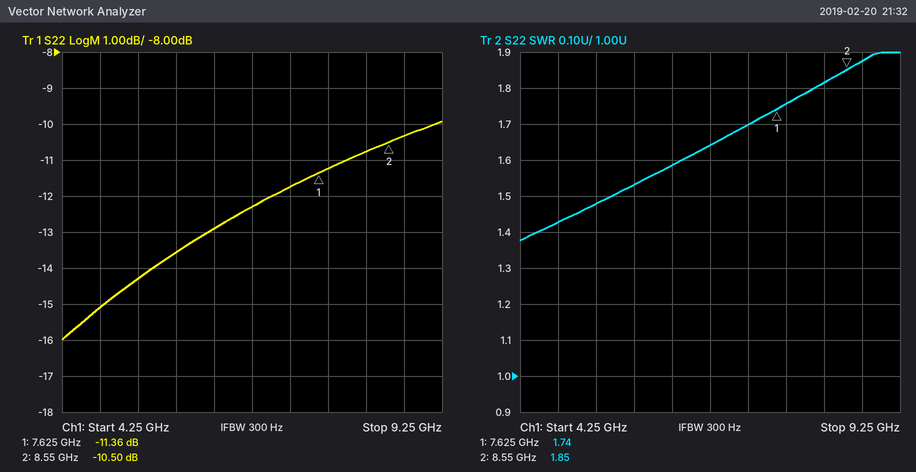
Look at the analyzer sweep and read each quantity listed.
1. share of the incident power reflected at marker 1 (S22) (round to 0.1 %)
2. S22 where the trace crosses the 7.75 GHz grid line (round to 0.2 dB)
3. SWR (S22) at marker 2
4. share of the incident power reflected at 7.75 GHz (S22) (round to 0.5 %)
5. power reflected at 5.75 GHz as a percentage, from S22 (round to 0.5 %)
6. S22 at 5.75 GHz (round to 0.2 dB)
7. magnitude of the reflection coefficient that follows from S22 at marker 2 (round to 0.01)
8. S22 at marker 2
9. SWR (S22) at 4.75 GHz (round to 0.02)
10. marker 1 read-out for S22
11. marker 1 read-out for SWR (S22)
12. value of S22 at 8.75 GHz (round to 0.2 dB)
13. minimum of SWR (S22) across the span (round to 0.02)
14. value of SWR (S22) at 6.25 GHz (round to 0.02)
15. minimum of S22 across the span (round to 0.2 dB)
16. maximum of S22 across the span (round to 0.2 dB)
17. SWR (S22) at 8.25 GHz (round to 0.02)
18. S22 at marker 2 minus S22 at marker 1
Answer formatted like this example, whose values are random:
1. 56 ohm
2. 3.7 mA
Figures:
1. 7.3 %
2. -11.2 dB
3. 1.85
4. 7.5 %
5. 4.5 %
6. -13.6 dB
7. 0.30
8. -10.50 dB
9. 1.42
10. -11.36 dB
11. 1.74
12. -10.4 dB
13. 1.38
14. 1.58
15. -16.0 dB
16. -10.0 dB
17. 1.82
18. 0.86 dB
